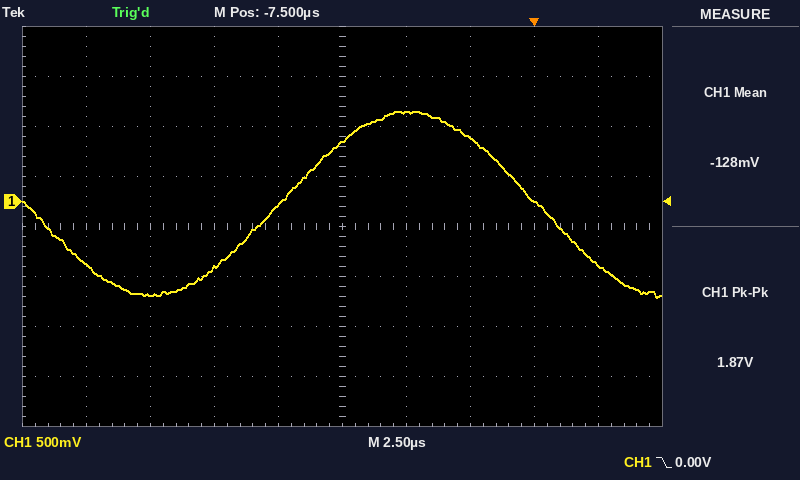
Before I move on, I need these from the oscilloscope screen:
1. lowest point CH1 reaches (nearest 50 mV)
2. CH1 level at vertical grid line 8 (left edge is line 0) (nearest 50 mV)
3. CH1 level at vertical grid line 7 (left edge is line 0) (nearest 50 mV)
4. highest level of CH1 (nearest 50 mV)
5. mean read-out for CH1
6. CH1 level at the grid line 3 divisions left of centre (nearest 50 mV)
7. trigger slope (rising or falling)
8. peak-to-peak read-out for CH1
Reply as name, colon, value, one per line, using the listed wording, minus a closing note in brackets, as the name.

lowest point CH1 reaches: -950 mV
CH1 level at vertical grid line 8 (left edge is line 0): 0 mV
CH1 level at vertical grid line 7 (left edge is line 0): 650 mV
highest level of CH1: 900 mV
mean read-out for CH1: -128 mV
CH1 level at the grid line 3 divisions left of centre: -950 mV
trigger slope: falling
peak-to-peak read-out for CH1: 1.87 V
